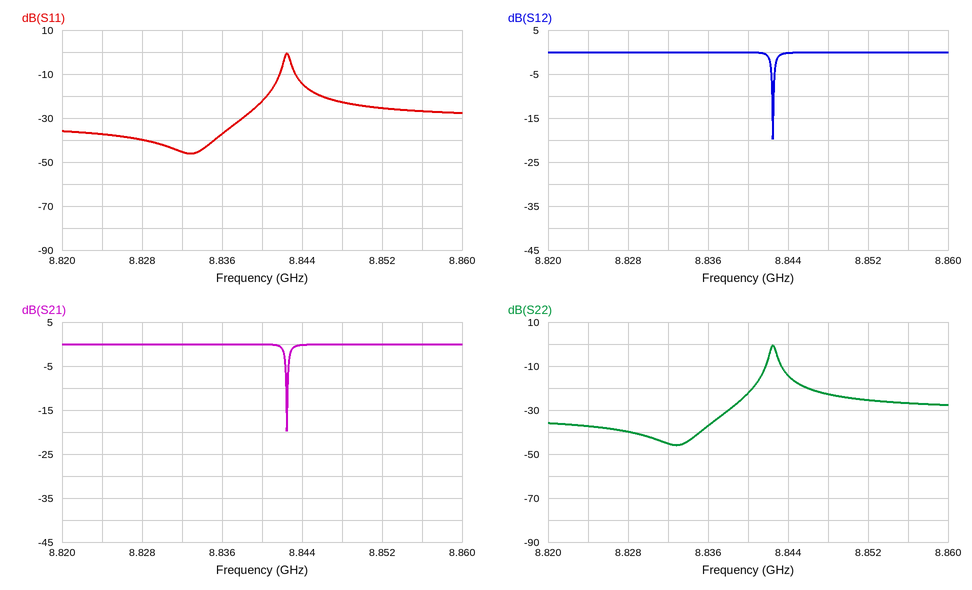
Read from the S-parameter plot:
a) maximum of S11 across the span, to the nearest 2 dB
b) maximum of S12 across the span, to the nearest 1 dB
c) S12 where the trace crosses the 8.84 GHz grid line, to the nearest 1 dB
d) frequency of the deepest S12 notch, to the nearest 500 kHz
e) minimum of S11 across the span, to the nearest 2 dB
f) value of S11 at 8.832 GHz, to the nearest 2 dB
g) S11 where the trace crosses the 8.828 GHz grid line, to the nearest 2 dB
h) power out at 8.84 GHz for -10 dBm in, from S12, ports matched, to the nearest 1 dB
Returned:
0 dB
0 dB
0 dB
8.8425 GHz
-46 dB
-46 dB
-40 dB
-10 dBm
